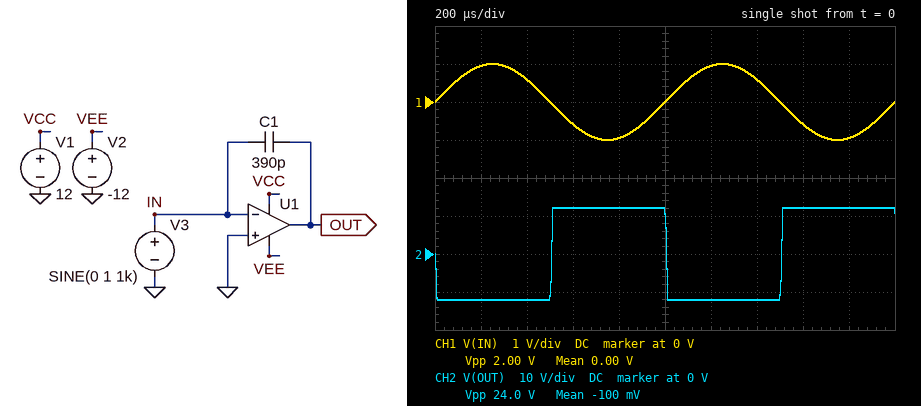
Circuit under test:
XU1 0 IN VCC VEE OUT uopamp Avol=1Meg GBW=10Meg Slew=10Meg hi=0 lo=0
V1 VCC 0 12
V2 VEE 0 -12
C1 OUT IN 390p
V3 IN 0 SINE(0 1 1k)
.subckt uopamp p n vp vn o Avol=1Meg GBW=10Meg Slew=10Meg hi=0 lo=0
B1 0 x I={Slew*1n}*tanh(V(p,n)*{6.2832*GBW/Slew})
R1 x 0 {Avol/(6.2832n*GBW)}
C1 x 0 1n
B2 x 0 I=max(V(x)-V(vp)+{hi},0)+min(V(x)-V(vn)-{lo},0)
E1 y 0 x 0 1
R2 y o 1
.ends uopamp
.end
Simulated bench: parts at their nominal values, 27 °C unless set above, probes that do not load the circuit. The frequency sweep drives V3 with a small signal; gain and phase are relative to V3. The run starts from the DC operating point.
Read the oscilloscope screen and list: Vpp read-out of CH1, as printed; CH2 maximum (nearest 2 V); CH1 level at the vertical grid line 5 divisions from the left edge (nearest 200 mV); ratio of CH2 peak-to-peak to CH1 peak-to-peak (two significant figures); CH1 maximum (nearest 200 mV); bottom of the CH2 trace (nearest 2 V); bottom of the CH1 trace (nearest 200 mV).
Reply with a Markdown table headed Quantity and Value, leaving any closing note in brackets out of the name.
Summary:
| Quantity | Value |
|---|---|
| Vpp read-out of CH1, as printed | 2.00 V |
| CH2 maximum | 12 V |
| CH1 level at the vertical grid line 5 divisions from the left edge | 0 V |
| ratio of CH2 peak-to-peak to CH1 peak-to-peak | 12 |
| CH1 maximum | 1.0 V |
| bottom of the CH2 trace | -12 V |
| bottom of the CH1 trace | -1.0 V |
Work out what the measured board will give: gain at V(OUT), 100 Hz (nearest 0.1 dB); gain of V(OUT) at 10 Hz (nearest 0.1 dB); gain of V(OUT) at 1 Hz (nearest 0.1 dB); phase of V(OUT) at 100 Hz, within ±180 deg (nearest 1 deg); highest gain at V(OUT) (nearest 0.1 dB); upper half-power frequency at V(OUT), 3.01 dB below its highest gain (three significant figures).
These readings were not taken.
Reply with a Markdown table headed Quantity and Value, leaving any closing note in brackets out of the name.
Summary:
| Quantity | Value |
|---|---|
| gain at V(OUT), 100 Hz | 100.0 dB |
| gain of V(OUT) at 10 Hz | 117.0 dB |
| gain of V(OUT) at 1 Hz | 120.0 dB |
| phase of V(OUT) at 100 Hz, within ±180 deg | 96 deg |
| highest gain at V(OUT) | 120.0 dB |
| upper half-power frequency at V(OUT), 3.01 dB below its highest gain | 10.0 Hz |
